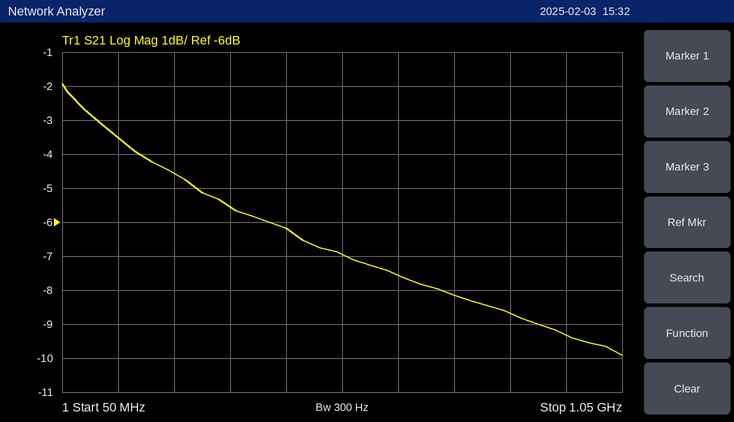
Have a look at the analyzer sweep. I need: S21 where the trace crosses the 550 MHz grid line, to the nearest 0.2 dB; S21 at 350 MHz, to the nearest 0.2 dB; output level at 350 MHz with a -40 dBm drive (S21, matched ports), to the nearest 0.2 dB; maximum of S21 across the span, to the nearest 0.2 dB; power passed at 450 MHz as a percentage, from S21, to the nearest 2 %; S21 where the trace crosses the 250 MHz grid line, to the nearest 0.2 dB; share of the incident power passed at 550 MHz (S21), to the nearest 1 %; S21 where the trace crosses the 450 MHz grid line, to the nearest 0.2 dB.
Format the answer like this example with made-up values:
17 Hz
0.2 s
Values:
-7.0 dB
-5.6 dB
-45.6 dBm
-2.0 dB
24 %
-4.6 dB
20 %
-6.2 dB
